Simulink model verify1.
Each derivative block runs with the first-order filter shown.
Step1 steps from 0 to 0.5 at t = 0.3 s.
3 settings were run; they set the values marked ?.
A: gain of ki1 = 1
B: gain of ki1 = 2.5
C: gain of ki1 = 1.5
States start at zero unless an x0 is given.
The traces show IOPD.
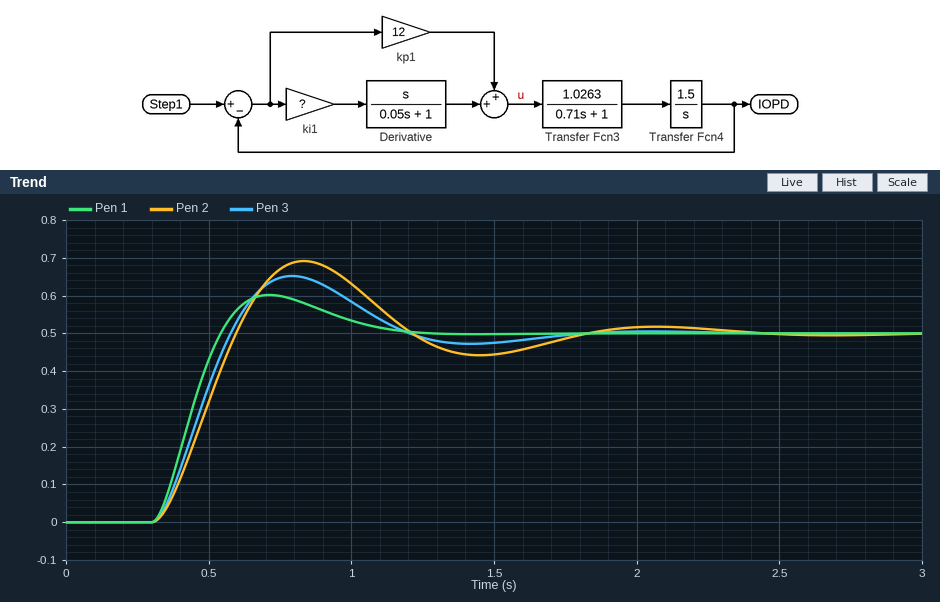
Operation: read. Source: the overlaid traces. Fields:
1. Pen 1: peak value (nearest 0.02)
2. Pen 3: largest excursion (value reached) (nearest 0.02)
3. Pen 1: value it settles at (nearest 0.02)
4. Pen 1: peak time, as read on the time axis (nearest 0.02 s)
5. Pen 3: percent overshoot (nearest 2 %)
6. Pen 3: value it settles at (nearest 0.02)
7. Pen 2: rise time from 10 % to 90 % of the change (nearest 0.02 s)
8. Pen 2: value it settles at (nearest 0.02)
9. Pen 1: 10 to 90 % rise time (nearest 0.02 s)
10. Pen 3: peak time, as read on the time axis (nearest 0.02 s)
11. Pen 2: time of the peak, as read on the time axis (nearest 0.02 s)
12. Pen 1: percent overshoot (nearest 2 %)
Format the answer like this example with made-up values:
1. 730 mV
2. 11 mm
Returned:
1. 0.60
2. 0.66
3. 0.50
4. 0.72 s
5. 30 %
6. 0.50
7. 0.20 s
8. 0.50
9. 0.16 s
10. 0.80 s
11. 0.84 s
12. 20 %
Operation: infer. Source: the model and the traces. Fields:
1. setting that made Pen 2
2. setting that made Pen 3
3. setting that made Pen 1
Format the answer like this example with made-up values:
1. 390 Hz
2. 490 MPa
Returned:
1. A
2. C
3. B
